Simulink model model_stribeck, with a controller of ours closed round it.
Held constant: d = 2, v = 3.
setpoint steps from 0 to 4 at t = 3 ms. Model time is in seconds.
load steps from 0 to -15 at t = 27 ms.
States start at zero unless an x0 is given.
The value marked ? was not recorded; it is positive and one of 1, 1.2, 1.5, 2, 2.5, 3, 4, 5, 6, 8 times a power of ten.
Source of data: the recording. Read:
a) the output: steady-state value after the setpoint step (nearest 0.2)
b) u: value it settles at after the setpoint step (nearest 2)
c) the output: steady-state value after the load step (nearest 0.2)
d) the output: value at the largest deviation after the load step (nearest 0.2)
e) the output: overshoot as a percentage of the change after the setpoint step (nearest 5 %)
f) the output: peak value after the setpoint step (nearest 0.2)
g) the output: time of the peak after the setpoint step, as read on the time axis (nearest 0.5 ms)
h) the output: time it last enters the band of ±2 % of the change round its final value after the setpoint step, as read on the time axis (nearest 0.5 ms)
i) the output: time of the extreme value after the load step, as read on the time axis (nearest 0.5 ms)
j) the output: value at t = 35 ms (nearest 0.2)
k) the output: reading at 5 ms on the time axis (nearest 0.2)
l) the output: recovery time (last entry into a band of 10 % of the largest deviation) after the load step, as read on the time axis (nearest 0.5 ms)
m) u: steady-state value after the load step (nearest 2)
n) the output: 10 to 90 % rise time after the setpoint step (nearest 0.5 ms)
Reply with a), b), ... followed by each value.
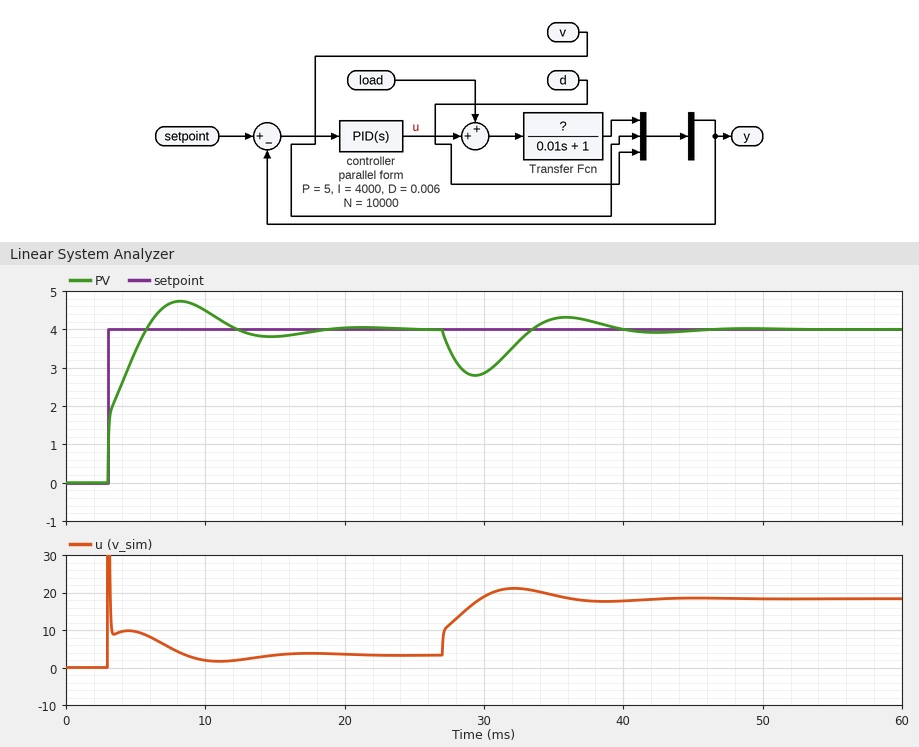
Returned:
a) 4.0
b) 4
c) 4.0
d) 2.8
e) 20 %
f) 4.8
g) 8.0 ms
h) 17.5 ms
i) 29.5 ms
j) 4.2
k) 3.4
l) 38.5 ms
m) 18
n) 2.0 ms
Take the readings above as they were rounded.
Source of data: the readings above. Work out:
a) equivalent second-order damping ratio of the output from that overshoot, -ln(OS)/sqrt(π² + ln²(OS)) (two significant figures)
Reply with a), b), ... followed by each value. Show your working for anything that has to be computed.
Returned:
a) ln(0.2) = -1.609; 1.609 / sqrt(9.870 + 2.590) = 0.46
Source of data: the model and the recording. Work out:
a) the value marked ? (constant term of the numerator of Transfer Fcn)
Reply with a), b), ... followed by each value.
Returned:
a) 1.2
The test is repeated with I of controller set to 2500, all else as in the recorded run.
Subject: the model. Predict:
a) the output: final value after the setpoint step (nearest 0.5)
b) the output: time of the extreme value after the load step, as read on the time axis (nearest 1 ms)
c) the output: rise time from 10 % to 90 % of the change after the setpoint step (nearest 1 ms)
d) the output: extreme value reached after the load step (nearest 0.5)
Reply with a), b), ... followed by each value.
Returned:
a) 4.0
b) 30 ms
c) 3 ms
d) 2.5
